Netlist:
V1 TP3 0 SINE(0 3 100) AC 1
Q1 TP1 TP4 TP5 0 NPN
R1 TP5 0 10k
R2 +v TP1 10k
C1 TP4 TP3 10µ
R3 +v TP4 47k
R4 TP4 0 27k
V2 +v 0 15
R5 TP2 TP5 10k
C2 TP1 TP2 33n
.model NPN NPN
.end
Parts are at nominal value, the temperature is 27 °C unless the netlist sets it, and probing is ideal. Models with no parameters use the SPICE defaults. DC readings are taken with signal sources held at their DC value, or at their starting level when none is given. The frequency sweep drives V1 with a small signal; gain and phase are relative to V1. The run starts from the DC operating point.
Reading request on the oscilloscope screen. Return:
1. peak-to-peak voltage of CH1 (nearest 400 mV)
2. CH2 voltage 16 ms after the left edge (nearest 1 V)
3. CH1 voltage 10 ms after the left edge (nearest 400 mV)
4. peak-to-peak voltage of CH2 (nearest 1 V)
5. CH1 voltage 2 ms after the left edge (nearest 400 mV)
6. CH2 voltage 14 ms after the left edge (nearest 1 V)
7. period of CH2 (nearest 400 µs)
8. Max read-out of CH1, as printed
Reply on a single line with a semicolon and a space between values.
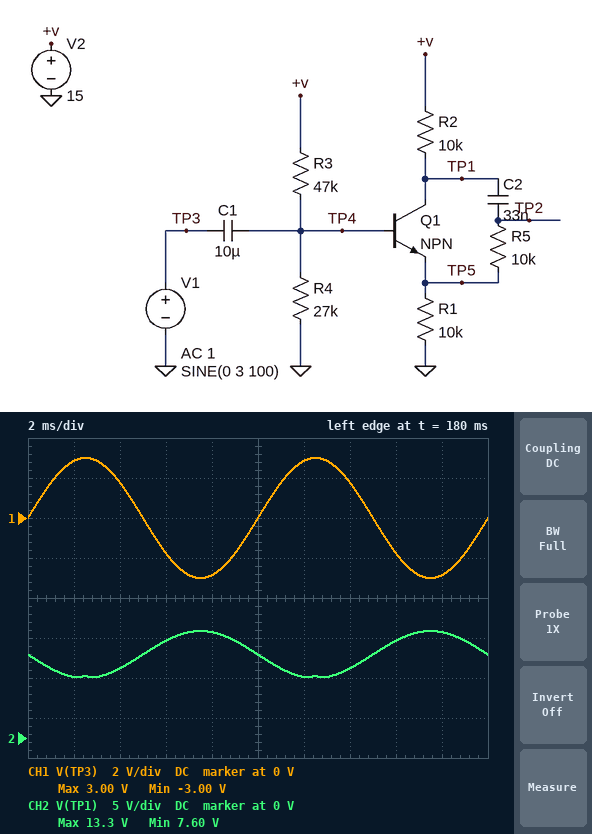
6.0 V; 12 V; 0 V; 6 V; 2.8 V; 9 V; 10.0 ms; 3.00 V
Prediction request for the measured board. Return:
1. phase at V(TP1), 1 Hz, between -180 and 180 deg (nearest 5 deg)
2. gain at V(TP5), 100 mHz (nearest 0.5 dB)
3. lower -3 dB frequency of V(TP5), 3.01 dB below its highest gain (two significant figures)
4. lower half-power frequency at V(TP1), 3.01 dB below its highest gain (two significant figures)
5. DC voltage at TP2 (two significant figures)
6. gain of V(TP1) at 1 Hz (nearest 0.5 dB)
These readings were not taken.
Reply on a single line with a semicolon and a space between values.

-135 deg; -19.5 dB; 940 mHz; 940 mHz; 4.6 V; -3.0 dB
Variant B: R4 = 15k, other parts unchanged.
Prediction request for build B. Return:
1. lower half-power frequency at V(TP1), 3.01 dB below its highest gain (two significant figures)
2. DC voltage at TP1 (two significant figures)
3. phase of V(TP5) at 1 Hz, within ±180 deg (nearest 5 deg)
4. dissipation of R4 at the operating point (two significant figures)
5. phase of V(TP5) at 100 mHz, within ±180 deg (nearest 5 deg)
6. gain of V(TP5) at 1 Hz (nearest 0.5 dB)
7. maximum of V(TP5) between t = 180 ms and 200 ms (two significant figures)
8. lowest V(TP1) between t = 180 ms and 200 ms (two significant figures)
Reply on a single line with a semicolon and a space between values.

1.4 Hz; 12 V; 55 deg; 860 µW; 85 deg; -5.0 dB; 5.8 V; 9.2 V
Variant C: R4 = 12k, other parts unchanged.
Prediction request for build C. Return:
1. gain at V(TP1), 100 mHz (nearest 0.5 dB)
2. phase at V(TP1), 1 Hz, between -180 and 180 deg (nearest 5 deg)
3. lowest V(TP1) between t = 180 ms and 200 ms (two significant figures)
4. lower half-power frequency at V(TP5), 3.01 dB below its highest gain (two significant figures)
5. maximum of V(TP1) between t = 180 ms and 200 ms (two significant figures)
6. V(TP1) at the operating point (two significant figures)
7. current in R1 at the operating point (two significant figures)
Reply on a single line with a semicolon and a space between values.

-24.5 dB; -120 deg; 9.8 V; 1.7 Hz; 15 V; 13 V; 230 µA
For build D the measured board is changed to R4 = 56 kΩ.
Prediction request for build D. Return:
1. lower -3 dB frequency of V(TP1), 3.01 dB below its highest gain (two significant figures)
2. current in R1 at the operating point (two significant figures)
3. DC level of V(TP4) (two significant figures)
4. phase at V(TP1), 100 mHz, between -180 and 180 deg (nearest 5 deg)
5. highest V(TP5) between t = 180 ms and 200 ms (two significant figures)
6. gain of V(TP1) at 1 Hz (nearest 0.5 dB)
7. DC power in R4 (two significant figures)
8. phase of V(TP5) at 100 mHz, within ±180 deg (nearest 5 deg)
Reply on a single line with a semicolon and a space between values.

640 mHz; 720 µA; 8.0 V; -100 deg; 9.0 V; -1.5 dB; 1.1 mW; 80 deg
